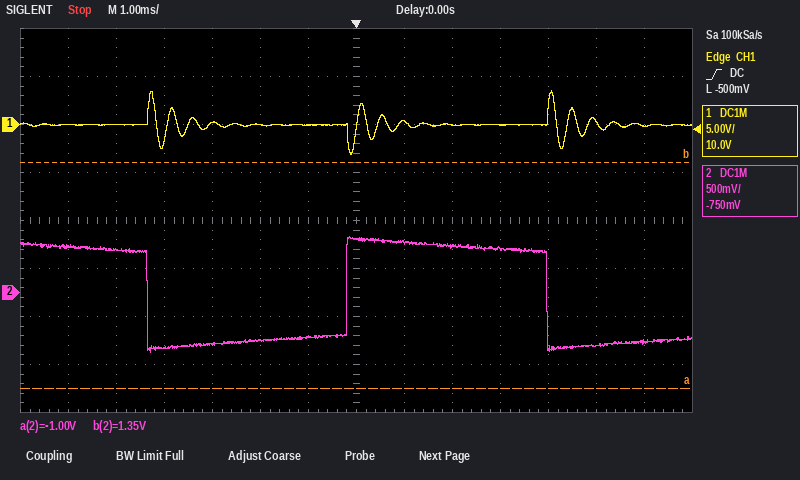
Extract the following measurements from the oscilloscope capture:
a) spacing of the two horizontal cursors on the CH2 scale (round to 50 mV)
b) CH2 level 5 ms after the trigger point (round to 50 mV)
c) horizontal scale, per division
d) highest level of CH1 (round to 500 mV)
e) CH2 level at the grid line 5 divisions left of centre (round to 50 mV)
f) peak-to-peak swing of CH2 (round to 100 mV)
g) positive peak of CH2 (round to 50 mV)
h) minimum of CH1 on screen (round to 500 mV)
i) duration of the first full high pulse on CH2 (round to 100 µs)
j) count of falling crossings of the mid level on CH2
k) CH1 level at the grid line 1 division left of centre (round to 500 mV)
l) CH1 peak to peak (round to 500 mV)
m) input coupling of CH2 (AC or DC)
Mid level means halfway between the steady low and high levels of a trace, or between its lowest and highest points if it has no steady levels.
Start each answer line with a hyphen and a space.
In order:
- 2.35 V
- -550 mV
- 1 ms
- 3.5 V
- 450 mV
- 1.20 V
- 600 mV
- -3.0 V
- 4.2 ms
- 2
- 0.0 V
- 6.5 V
- DC
